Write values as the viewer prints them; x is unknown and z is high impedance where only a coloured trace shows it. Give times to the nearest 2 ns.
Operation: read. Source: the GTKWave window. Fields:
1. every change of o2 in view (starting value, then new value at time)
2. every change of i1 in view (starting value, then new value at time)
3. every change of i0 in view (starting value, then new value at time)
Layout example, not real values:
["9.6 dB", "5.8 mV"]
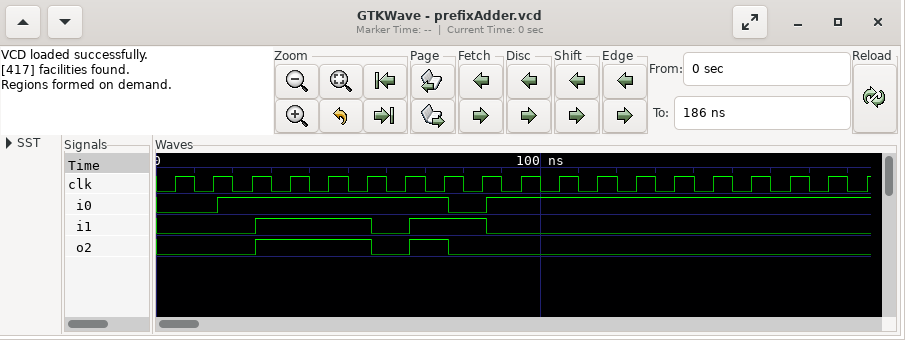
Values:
["0, 1 at 26 ns, 0 at 56 ns, 1 at 66 ns, 0 at 76 ns", "0, 1 at 26 ns, 0 at 56 ns, 1 at 66 ns, 0 at 86 ns", "0, 1 at 16 ns, 0 at 76 ns, 1 at 86 ns"]
